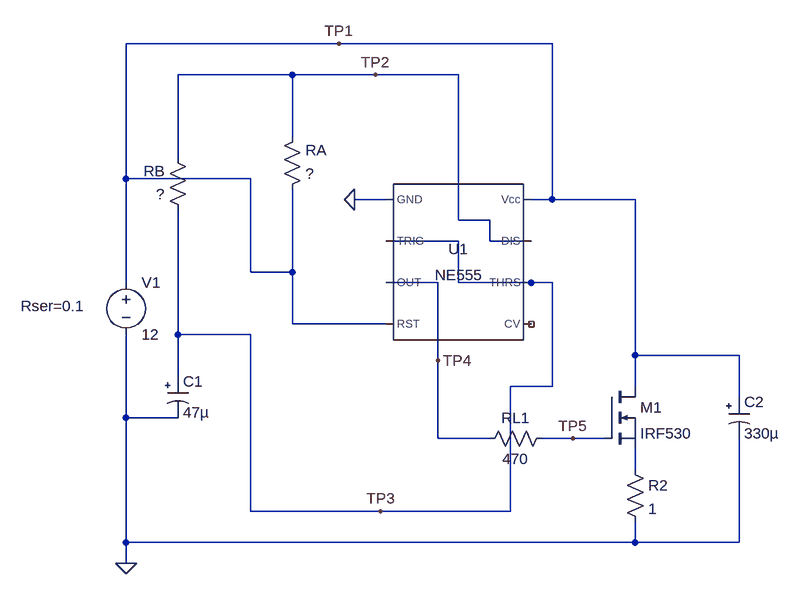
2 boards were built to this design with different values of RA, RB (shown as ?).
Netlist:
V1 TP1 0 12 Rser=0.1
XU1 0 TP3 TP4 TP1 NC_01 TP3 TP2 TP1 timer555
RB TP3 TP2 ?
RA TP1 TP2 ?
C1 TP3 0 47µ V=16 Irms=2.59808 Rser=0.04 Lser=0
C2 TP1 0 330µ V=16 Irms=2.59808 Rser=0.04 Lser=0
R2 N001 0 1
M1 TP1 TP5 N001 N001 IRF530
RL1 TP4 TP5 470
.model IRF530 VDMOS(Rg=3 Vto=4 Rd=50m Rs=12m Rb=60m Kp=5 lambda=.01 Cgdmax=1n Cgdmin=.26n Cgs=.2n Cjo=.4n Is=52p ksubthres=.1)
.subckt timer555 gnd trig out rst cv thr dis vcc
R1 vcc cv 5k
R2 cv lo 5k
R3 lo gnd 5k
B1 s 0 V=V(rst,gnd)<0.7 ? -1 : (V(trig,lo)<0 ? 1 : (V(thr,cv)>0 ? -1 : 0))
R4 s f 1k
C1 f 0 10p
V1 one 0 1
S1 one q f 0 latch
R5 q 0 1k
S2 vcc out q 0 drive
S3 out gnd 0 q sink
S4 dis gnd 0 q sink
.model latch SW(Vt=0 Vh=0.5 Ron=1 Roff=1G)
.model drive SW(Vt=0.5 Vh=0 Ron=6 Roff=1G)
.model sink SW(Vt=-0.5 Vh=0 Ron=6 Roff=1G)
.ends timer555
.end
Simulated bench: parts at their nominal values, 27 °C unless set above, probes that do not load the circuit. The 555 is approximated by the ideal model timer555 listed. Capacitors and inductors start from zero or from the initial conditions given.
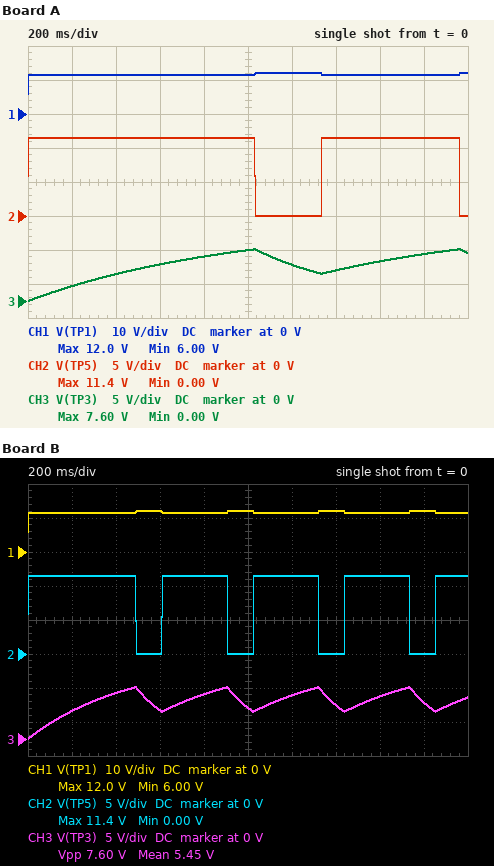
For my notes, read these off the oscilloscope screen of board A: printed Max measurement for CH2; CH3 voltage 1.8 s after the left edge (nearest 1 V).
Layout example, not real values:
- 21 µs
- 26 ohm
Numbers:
- 11.4 V
- 7 V
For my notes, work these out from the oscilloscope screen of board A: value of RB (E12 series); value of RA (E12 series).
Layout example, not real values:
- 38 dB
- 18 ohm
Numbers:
- 10 kΩ
- 10 kΩ
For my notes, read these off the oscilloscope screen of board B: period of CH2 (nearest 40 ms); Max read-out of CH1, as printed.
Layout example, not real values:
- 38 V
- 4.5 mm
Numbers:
- 400 ms
- 12.0 V
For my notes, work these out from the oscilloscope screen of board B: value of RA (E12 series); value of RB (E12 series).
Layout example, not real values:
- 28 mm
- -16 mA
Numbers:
- 5.6 kΩ
- 3.9 kΩ
